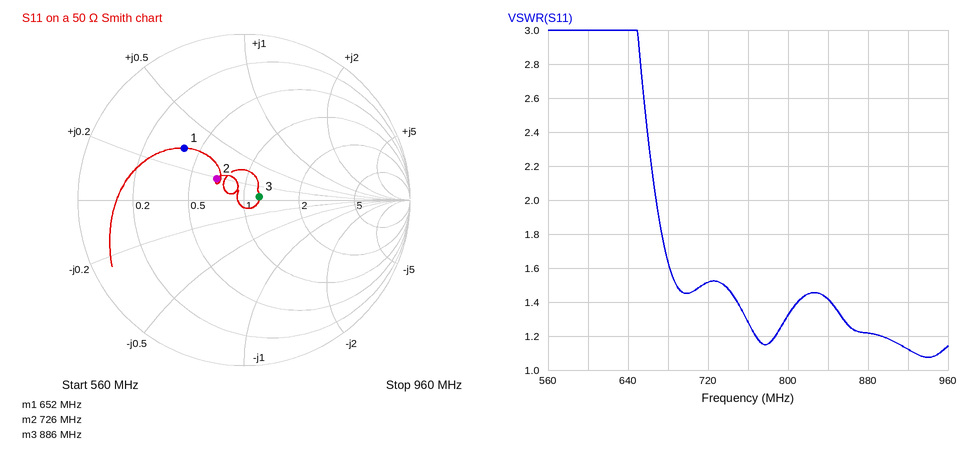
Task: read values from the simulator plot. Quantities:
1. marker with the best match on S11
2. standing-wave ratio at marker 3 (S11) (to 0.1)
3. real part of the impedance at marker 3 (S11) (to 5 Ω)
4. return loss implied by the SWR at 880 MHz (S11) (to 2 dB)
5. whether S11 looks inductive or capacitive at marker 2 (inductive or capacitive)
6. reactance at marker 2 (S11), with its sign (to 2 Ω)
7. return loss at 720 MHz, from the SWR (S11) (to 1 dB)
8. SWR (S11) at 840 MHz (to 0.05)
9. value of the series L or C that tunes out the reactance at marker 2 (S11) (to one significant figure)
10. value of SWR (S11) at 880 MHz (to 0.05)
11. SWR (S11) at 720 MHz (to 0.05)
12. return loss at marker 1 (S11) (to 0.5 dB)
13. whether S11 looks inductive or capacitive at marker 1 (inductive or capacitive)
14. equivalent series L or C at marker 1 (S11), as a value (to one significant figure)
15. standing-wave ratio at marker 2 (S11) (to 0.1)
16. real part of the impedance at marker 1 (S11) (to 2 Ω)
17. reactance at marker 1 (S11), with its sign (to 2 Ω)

marker 3
1.2
60 Ω
20 dB
inductive
+10 Ω
14 dB
1.40
20 pF
1.20
1.50
6.5 dB
inductive
4 nH
1.5
20 Ω
+16 Ω
